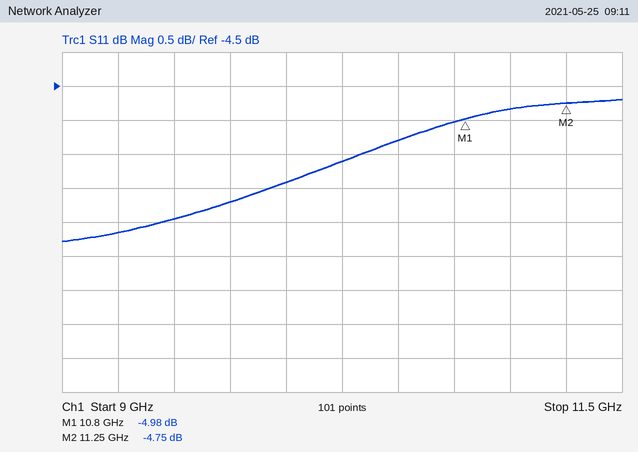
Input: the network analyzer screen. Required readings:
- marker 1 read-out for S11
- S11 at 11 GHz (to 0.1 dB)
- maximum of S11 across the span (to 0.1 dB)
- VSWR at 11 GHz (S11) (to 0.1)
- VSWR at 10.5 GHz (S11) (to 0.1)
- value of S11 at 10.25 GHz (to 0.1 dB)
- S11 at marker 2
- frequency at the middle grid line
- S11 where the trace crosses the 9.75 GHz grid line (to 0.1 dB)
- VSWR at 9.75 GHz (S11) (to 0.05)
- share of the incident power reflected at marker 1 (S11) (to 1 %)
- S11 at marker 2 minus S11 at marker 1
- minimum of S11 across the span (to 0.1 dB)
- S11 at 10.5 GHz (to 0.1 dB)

-4.98 dB
-4.8 dB
-4.7 dB
3.7
3.4
-5.6 dB
-4.75 dB
10.25 GHz
-6.2 dB
2.90
32 %
0.23 dB
-6.8 dB
-5.3 dB
